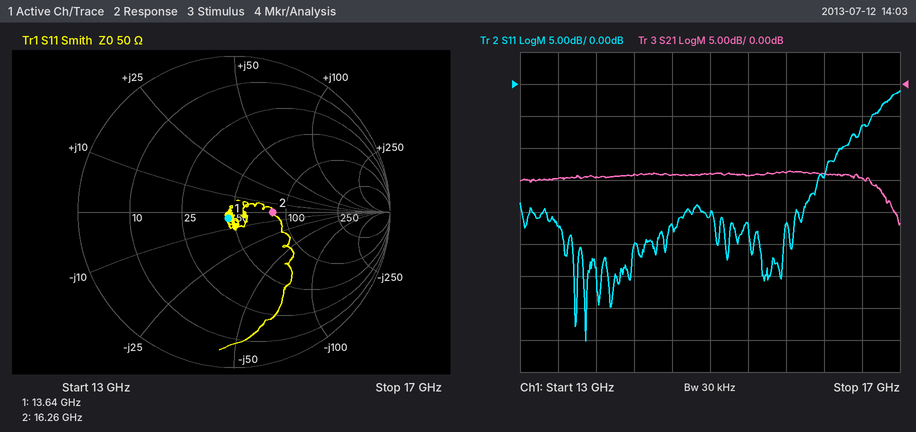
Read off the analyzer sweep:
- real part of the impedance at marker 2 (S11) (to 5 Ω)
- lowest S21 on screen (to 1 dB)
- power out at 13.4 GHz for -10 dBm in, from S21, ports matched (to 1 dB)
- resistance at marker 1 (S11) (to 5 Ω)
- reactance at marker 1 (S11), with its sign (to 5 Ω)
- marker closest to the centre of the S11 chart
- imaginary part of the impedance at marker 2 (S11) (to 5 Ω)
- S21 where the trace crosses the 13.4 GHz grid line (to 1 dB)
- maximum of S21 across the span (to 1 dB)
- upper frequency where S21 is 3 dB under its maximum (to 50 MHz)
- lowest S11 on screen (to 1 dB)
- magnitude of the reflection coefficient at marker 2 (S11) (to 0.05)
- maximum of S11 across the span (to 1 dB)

85 Ω
-22 dB
-25 dBm
45 Ω
-5 Ω
marker 1
0 Ω
-15 dB
-14 dB
16.80 GHz
-40 dB
0.25
-1 dB
